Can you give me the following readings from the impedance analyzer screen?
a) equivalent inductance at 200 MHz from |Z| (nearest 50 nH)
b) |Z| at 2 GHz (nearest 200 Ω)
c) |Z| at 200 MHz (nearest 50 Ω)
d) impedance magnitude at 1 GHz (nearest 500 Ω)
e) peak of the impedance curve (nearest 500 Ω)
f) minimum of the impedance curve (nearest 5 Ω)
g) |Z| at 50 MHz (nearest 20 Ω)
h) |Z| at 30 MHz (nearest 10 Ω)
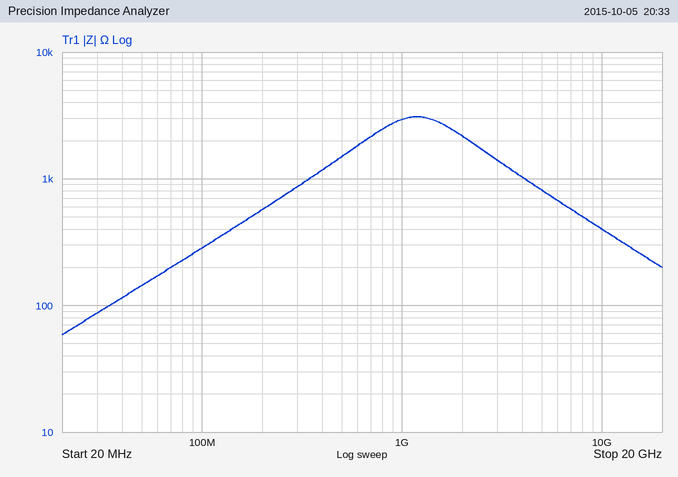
450 nH
2.2 kΩ
550 Ω
3.0 kΩ
3.0 kΩ
60 Ω
140 Ω
90 Ω
